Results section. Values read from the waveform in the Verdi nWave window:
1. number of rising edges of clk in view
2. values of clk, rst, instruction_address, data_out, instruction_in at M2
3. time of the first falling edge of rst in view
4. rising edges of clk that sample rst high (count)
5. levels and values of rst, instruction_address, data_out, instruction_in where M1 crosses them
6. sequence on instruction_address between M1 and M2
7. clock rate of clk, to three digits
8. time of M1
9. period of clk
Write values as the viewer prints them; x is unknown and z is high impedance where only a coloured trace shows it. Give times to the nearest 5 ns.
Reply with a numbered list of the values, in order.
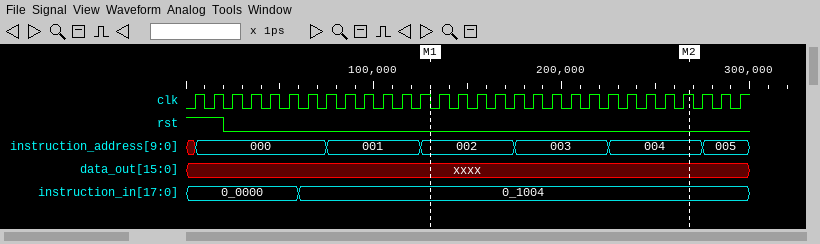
1. 30
2. clk=1, rst=0, instruction_address=004, data_out=xxxx, instruction_in=0_1004
3. 20 ns
4. 2
5. rst=0, instruction_address=002, data_out=xxxx, instruction_in=0_1004
6. 002, 003, 004
7. 100 MHz
8. 130 ns
9. 10 ns
